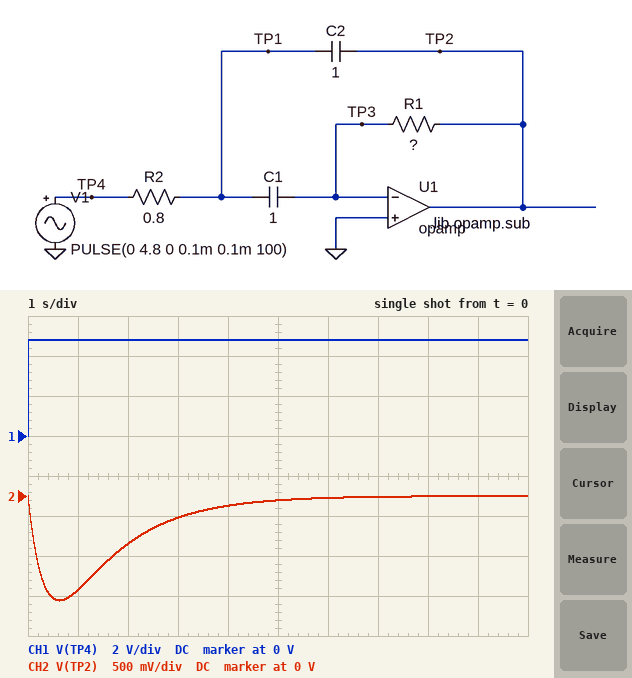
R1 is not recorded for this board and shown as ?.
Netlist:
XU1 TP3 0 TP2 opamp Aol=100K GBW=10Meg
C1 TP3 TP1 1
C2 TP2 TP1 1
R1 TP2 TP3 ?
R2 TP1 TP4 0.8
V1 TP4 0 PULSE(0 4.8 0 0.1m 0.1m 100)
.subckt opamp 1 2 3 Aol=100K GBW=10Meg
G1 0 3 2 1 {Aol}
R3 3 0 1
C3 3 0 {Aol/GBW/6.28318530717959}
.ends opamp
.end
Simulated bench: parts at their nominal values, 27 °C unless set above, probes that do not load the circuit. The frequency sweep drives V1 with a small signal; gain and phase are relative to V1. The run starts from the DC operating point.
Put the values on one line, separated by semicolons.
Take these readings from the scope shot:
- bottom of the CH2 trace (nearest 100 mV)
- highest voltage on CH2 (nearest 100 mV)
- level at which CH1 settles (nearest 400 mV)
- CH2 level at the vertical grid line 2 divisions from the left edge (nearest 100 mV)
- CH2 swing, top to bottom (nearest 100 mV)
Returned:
-1.3 V; 0 V; 4.8 V; -600 mV; 1.3 V
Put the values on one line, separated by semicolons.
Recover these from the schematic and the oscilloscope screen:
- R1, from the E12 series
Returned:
0.56 Ω
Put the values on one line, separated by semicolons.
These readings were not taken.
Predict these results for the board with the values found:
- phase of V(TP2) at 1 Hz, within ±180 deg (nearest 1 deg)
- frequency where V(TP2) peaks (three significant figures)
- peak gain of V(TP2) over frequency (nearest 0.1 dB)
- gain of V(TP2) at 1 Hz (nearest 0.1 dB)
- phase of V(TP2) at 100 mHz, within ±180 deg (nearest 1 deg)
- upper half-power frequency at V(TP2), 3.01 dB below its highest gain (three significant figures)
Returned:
121 deg; 238 mHz; -9.1 dB; -14.9 dB; -141 deg; 655 mHz
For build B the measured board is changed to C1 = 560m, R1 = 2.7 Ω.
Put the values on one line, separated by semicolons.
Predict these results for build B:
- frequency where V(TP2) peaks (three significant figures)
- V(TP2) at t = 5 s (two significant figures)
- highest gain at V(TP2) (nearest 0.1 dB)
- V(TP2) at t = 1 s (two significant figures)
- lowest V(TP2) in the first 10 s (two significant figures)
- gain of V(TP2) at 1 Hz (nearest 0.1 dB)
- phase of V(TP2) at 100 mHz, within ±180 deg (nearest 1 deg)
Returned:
145 mHz; 340 mV; 1.7 dB; -3.3 V; -3.4 V; -14.0 dB; -146 deg
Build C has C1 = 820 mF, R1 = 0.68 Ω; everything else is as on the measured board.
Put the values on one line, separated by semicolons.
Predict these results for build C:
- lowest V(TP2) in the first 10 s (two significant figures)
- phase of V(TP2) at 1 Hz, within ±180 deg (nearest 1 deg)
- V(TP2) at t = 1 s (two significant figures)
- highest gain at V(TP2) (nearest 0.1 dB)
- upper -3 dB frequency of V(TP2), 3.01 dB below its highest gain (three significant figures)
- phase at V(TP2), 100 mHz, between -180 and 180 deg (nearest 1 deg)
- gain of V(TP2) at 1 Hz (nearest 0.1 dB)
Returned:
-1.4 V; 119 deg; -1.3 V; -8.3 dB; 612 mHz; -138 deg; -14.7 dB
